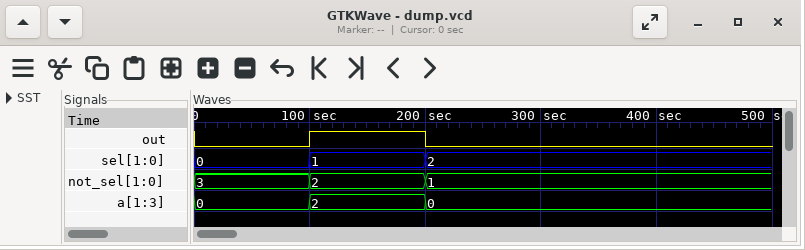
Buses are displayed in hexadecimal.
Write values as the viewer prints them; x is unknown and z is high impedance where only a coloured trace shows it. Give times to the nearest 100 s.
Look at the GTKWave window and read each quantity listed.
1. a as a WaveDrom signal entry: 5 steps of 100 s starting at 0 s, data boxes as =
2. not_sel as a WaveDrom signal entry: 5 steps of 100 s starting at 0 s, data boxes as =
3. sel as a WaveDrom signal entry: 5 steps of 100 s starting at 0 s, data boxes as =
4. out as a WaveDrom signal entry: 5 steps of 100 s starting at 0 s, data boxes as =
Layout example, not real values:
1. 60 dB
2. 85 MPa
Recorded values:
1. {name: 'a', wave: '===..', data: '0 2 0'}
2. {name: 'not_sel', wave: '===..', data: '3 2 1'}
3. {name: 'sel', wave: '===..', data: '0 1 2'}
4. {name: 'out', wave: '010..'}
